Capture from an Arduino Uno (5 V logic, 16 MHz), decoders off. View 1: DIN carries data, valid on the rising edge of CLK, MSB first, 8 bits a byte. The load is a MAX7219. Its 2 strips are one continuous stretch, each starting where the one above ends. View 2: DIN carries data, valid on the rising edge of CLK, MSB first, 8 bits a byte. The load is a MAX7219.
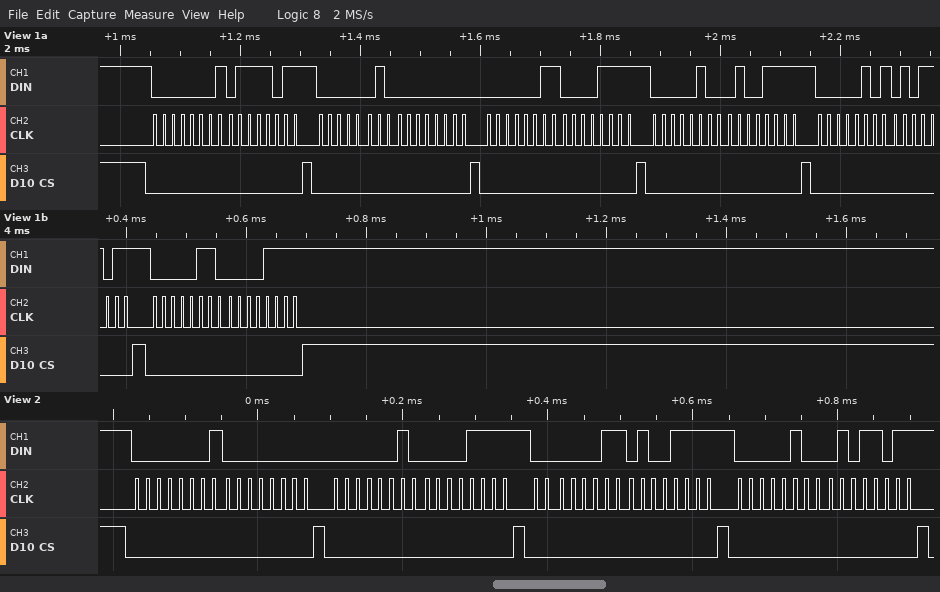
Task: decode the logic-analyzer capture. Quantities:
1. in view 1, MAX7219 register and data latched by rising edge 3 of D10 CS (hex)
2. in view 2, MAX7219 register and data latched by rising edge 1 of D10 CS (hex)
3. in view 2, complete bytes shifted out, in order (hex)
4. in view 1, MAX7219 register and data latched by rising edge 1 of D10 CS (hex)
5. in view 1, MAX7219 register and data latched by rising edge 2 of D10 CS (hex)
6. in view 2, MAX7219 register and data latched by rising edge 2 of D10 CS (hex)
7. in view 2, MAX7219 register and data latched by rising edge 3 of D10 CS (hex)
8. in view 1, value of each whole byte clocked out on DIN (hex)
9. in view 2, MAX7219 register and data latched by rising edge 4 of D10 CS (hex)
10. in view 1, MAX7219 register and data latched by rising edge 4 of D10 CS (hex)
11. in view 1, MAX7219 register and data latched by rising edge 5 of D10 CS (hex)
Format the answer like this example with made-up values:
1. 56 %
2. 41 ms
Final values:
1. register 0x3, data 0x0F
2. register 0x1, data 0x00
3. 0x01 0x00 0x02 0x0F 0x03 0x4F 0x04 0x5B
4. register 0x1, data 0x7B
5. register 0x2, data 0x00
6. register 0x2, data 0x0F
7. register 0x3, data 0x4F
8. 0x01 0x7B 0x02 0x00 0x03 0x0F 0x04 0x4F 0x05 0x5B 0x06 0x0F
9. register 0x4, data 0x5B
10. register 0x4, data 0x4F
11. register 0x5, data 0x5B
